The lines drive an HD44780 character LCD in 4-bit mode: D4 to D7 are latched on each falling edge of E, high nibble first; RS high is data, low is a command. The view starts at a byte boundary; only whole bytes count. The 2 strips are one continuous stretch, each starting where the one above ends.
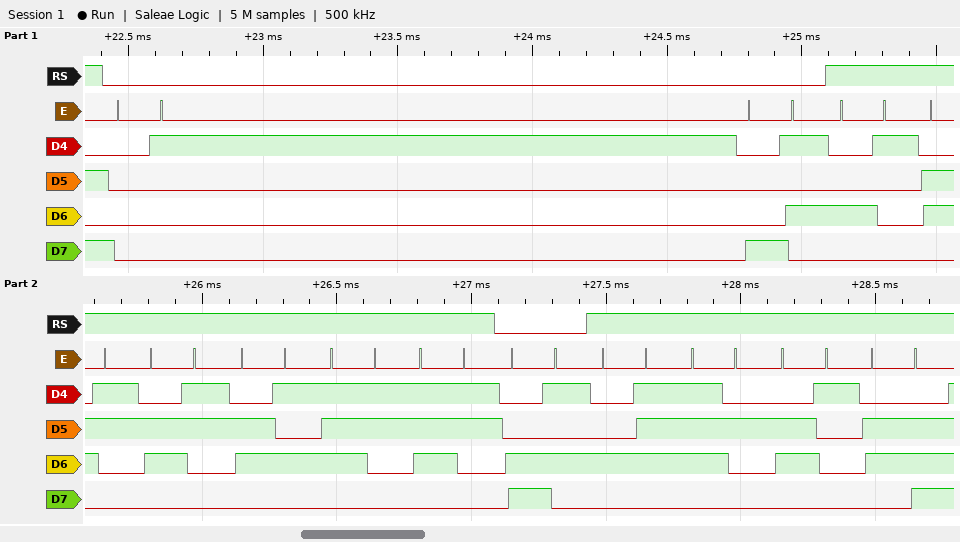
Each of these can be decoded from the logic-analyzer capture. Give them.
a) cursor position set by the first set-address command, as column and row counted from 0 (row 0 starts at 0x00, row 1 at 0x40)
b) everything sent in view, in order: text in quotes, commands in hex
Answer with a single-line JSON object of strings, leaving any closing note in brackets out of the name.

{"cursor position set by the first set-address command, as column and row counted from 0": "column 5, row 0", "everything sent in view, in order: text in quotes, commands in hex": "0x01 0x85 \"Access\" 0xC5 \"Gran\""}
